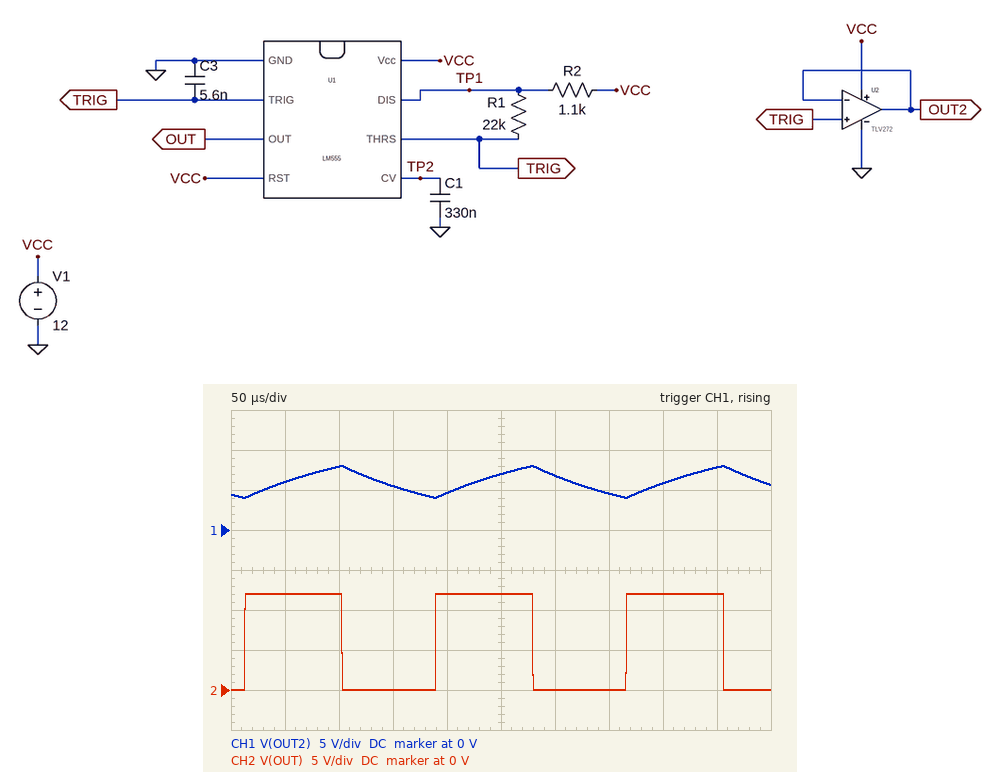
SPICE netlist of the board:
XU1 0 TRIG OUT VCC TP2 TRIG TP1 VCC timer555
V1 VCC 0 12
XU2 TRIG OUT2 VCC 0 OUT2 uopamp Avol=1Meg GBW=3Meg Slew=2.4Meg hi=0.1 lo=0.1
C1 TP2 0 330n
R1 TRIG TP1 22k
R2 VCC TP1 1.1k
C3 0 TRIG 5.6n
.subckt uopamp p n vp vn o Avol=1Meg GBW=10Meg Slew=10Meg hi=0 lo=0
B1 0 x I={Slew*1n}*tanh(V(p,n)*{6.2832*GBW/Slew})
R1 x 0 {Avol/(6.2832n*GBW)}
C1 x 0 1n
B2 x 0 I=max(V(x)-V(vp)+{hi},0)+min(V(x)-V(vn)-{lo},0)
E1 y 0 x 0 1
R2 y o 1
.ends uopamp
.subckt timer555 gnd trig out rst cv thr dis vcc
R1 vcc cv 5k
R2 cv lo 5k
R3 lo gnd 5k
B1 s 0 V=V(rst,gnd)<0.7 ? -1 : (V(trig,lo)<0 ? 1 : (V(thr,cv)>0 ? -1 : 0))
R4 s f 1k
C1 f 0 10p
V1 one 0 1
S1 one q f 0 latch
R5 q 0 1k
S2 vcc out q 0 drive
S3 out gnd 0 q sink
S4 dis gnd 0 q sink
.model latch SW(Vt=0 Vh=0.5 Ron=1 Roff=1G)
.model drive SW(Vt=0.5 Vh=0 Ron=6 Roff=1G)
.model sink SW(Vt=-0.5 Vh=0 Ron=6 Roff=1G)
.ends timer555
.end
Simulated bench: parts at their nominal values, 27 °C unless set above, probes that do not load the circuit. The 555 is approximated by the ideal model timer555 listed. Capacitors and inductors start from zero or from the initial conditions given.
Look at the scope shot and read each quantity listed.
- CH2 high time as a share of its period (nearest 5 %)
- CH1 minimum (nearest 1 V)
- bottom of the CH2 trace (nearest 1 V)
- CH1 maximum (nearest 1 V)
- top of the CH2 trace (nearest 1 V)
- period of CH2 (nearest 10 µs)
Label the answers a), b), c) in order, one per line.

a) 50 %
b) 4 V
c) 0 V
d) 8 V
e) 12 V
f) 180 µs
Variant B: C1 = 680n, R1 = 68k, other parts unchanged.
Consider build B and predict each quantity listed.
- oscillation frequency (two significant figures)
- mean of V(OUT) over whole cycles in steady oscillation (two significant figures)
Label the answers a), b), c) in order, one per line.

a) 1.9 kHz
b) 5.9 V
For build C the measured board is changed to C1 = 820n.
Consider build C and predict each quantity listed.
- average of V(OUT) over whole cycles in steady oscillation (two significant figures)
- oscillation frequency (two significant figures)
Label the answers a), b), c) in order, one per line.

a) 5.9 V
b) 5.9 kHz
